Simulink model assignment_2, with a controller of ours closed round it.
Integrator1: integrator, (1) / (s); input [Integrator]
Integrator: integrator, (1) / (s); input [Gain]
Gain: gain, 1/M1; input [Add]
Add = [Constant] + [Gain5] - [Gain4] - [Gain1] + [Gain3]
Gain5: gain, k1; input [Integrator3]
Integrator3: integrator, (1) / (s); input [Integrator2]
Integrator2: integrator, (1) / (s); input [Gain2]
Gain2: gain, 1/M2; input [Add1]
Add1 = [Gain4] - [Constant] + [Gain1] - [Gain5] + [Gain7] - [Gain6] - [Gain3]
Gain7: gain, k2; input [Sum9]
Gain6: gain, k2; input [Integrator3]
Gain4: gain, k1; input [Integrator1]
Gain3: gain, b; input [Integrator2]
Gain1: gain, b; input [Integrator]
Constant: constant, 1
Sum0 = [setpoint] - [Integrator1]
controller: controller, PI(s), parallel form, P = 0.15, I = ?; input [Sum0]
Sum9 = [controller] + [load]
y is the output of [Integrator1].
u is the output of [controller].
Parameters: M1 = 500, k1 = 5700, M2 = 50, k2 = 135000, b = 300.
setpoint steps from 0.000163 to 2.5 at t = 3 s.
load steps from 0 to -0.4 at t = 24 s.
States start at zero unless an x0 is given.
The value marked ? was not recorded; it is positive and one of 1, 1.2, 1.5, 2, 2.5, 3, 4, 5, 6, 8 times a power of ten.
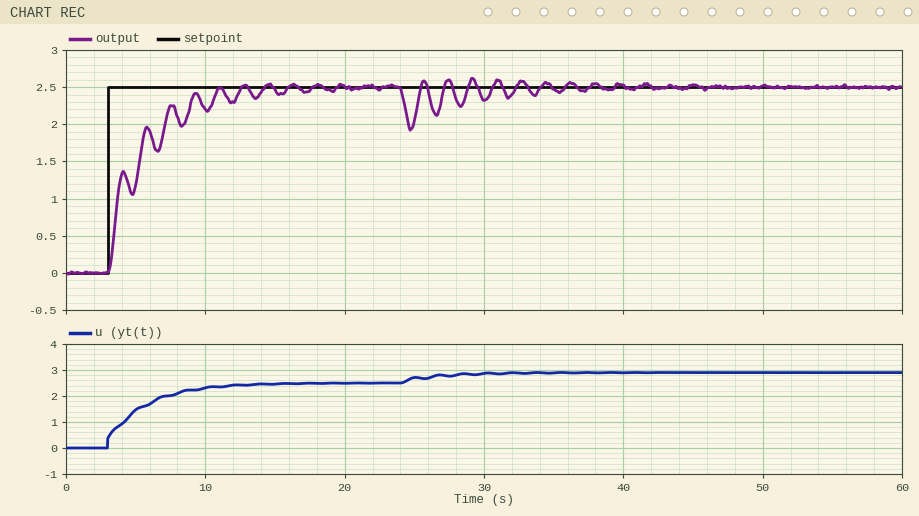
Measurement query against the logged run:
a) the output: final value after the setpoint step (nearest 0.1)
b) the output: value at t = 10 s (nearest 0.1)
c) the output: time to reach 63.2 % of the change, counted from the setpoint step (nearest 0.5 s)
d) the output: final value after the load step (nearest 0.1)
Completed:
2.5
2.2
2.5 s
2.5
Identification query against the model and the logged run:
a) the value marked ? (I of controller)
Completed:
0.4
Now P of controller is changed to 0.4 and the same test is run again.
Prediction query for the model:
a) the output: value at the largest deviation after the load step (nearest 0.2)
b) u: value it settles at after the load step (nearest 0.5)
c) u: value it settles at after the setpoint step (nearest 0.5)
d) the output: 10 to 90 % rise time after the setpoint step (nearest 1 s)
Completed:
2.0
3.0
2.5
5 s
